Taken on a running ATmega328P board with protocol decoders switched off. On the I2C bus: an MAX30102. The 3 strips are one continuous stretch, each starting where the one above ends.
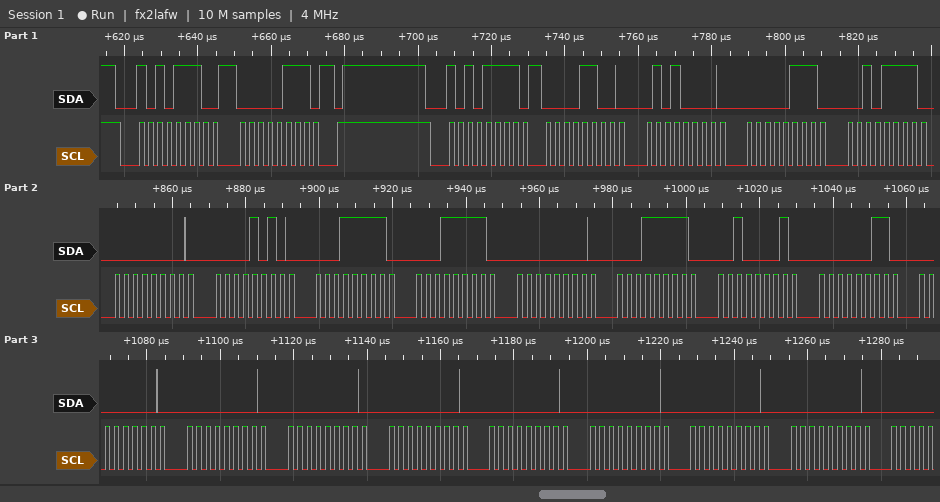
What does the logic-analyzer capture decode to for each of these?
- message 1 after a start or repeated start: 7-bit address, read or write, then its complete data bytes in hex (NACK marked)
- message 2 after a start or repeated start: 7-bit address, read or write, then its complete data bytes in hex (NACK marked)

0x57 write: 07
0x57 read: 0C 50 07 2F 00 0A 1F 1F 00 1F 21 03 00 00 00 00 00 00 00 00
